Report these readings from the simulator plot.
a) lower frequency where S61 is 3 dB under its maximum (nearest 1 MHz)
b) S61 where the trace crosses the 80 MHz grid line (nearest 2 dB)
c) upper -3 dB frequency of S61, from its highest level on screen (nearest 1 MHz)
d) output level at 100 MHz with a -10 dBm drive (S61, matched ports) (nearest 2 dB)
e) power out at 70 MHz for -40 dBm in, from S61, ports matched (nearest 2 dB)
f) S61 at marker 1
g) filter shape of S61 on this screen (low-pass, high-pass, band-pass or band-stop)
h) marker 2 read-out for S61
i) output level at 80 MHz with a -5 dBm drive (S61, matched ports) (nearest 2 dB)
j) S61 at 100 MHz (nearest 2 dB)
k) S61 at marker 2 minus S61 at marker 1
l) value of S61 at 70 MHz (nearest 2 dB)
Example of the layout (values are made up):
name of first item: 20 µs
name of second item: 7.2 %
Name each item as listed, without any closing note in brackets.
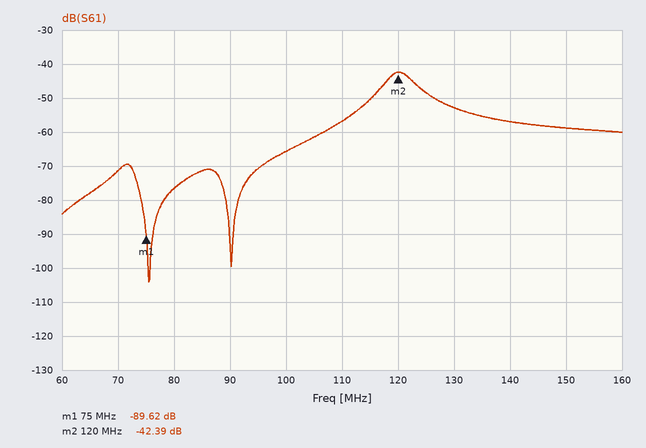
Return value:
lower frequency where S61 is 3 dB under its maximum: 118 MHz
S61 where the trace crosses the 80 MHz grid line: -76 dB
upper -3 dB frequency of S61, from its highest level on screen: 123 MHz
output level at 100 MHz with a -10 dBm drive (S61, matched ports): -76 dBm
power out at 70 MHz for -40 dBm in, from S61, ports matched: -112 dBm
S61 at marker 1: -89.62 dB
filter shape of S61 on this screen: band-pass
marker 2 read-out for S61: -42.39 dB
output level at 80 MHz with a -5 dBm drive (S61, matched ports): -82 dBm
S61 at 100 MHz: -66 dB
S61 at marker 2 minus S61 at marker 1: 47.23 dB
value of S61 at 70 MHz: -72 dB
